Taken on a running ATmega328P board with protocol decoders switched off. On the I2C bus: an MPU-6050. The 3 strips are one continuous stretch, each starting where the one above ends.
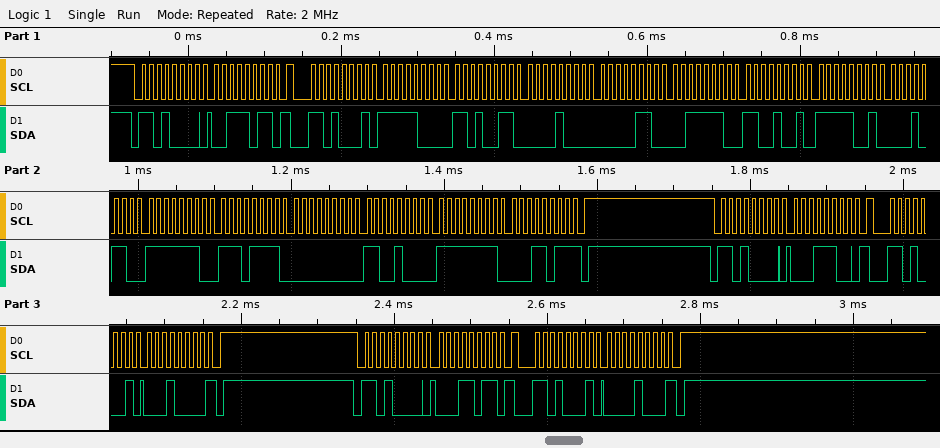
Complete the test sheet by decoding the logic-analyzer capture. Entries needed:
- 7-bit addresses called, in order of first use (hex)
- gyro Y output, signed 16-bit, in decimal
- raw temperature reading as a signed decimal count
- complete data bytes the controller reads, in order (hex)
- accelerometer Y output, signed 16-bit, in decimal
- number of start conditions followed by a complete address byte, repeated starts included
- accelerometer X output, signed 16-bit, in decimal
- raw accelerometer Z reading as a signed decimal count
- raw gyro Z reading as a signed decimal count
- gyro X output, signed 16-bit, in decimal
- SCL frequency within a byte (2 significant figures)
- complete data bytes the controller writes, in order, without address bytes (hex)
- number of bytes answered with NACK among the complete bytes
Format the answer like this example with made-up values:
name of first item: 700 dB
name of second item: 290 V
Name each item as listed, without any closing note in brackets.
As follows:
7-bit addresses called, in order of first use: 0x68
gyro Y output, signed 16-bit, in decimal: 200
raw temperature reading as a signed decimal count: -1770
complete data bytes the controller reads, in order: F8 D3 08 06 3E C9 F9 16 FE EF 00 C8 FF 1B 10 08
accelerometer Y output, signed 16-bit, in decimal: 2054
number of start conditions followed by a complete address byte, repeated starts included: 6
accelerometer X output, signed 16-bit, in decimal: -1837
raw accelerometer Z reading as a signed decimal count: 16073
raw gyro Z reading as a signed decimal count: -229
gyro X output, signed 16-bit, in decimal: -273
SCL frequency within a byte: 100 kHz
complete data bytes the controller writes, in order, without address bytes: 3B 1C 1B
number of bytes answered with NACK among the complete bytes: 3
